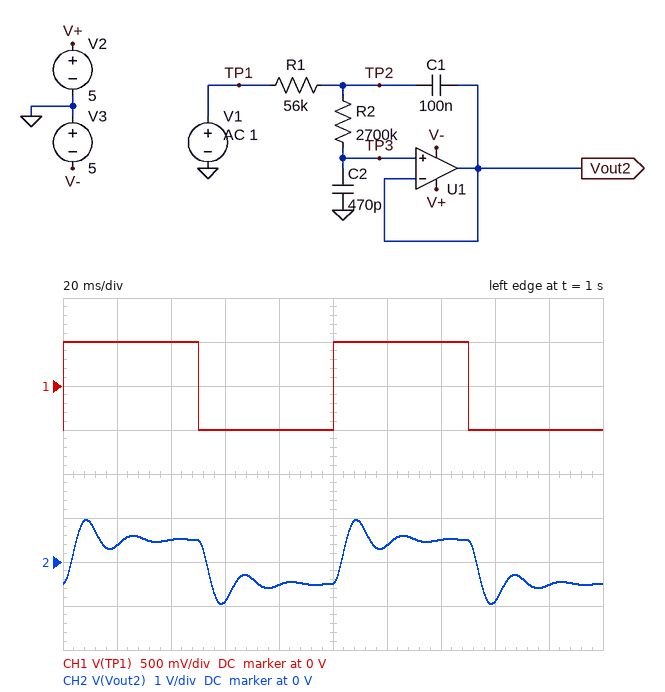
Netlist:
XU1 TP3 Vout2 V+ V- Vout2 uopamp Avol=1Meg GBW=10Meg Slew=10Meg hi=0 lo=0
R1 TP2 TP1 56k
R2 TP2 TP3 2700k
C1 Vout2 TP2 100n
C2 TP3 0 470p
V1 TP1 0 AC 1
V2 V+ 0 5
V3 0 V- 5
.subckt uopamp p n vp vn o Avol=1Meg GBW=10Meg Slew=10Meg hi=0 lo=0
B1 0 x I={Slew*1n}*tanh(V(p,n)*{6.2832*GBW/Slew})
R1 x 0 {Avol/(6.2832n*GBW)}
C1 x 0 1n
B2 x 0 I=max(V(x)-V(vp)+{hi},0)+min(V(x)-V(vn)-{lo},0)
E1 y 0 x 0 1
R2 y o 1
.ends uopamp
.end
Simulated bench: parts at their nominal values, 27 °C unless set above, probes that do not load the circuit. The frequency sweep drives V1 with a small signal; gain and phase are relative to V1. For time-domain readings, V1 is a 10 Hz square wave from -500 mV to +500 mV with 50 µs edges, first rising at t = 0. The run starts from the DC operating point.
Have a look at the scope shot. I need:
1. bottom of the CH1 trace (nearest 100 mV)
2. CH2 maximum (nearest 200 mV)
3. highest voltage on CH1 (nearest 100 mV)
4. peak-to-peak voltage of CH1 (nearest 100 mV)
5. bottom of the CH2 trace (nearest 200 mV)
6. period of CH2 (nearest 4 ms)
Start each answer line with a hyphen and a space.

- -500 mV
- 1.0 V
- 500 mV
- 1.0 V
- -1.0 V
- 100 ms
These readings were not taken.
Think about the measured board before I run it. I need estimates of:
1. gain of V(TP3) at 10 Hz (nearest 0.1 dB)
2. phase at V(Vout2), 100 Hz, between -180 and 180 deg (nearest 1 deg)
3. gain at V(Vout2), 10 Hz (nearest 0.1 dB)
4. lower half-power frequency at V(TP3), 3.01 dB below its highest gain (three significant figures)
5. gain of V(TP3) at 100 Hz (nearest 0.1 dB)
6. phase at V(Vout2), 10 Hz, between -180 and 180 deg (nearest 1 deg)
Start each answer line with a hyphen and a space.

- 0.2 dB
- -156 deg
- 0.2 dB
- 38.3 Hz
- -5.9 dB
- -5 deg
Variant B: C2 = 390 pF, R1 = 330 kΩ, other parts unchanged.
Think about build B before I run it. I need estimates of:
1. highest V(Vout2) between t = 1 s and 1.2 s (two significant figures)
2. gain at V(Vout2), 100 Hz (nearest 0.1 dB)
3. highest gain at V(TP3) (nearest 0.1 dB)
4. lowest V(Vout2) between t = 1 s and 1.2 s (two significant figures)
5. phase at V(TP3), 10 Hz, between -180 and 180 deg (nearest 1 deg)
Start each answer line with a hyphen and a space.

- 1.3 V
- -22.1 dB
- 14.0 dB
- -1.3 V
- -5 deg
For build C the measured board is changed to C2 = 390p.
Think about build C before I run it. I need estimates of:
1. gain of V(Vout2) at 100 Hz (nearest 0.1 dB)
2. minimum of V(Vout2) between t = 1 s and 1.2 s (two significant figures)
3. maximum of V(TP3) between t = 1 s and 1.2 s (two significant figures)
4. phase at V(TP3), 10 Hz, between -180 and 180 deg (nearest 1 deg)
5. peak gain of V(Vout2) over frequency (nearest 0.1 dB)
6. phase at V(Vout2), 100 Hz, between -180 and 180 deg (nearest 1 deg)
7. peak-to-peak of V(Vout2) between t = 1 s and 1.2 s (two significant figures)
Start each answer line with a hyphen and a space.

- -3.5 dB
- -990 mV
- 990 mV
- -4 deg
- 7.3 dB
- -153 deg
- 2.0 V
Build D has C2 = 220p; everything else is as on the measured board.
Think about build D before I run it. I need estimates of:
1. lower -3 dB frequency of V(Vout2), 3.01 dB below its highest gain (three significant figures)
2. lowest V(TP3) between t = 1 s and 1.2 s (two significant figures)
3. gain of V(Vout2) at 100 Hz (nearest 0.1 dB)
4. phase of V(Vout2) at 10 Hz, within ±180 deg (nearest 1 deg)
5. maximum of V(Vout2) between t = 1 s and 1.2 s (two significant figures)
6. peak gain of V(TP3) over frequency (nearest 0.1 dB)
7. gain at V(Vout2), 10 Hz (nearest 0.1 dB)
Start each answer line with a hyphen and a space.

- 68.5 Hz
- -1.1 V
- 6.1 dB
- -2 deg
- 1.1 V
- 9.7 dB
- 0.1 dB
